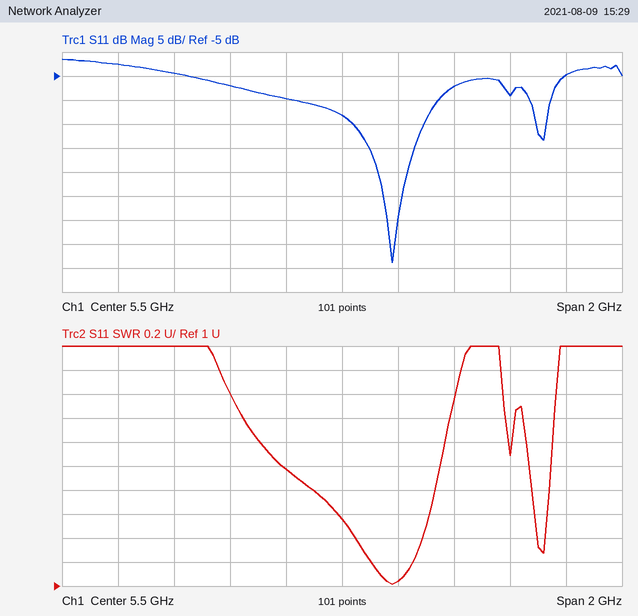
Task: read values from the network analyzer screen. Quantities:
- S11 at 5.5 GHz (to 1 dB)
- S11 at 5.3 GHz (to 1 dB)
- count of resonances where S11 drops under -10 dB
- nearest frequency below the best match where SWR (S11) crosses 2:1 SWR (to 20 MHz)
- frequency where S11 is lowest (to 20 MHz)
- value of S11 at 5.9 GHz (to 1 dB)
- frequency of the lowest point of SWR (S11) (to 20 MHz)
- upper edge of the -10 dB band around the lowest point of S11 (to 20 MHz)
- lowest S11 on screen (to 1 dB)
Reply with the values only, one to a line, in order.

-13 dB
-10 dB
2
5.28 GHz
5.68 GHz
-7 dB
5.68 GHz
5.84 GHz
-44 dB
